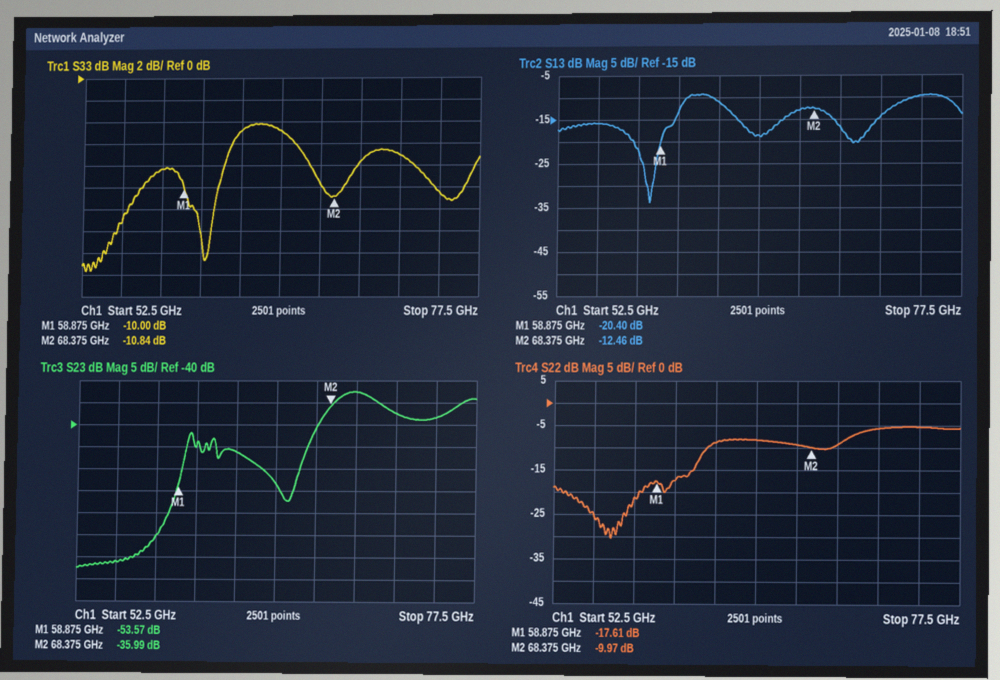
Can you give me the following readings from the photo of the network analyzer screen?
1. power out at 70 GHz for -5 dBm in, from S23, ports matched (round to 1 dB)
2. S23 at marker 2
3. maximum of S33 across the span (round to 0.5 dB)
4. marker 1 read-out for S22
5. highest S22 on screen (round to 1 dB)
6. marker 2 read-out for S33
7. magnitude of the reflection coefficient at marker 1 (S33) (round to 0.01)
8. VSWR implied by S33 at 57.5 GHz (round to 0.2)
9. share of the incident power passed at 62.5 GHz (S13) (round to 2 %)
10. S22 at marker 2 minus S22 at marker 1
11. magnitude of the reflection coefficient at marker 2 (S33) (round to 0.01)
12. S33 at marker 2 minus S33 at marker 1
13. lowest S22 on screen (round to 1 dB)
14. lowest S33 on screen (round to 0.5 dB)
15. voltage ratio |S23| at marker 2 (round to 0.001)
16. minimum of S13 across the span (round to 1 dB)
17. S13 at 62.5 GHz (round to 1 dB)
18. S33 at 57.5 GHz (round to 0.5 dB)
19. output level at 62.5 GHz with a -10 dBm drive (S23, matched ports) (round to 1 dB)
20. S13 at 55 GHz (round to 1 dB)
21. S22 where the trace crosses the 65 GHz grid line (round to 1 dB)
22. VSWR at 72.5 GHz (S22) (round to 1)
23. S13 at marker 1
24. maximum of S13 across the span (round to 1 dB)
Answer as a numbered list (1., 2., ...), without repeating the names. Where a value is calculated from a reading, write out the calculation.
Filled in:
1. -5 dBm + (-33 dB) = -38 dBm
2. -35.99 dB
3. -4.0 dB
4. -17.61 dB
5. -5 dB
6. -10.84 dB
7. 10^(-10/20) ≈ 0.32
8. |Γ| = 10^(-8.5/20) = 0.3758; VSWR = (1 + 0.3758)/(1 − 0.3758) ≈ 2.2
9. 10^(-11/10) ≈ 8 %
10. -9.97 − (-17.61) = 7.64 dB
11. 10^(-10.84/20) ≈ 0.29
12. -10.84 − (-10) = -0.84 dB
13. -30 dB
14. -17.5 dB
15. 10^(-35.99/20) ≈ 0.016
16. -34 dB
17. -11 dB
18. -8.5 dB
19. -10 dBm + (-46 dB) = -56 dBm
20. -16 dB
21. -8 dB
22. |Γ| = 10^(-6/20) = 0.5012; VSWR = (1 + 0.5012)/(1 − 0.5012) ≈ 3
23. -20.40 dB
24. -9 dB
